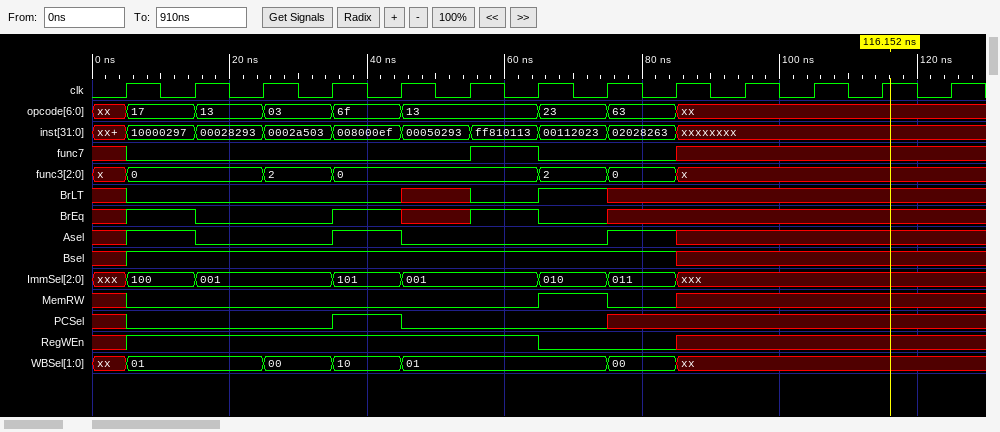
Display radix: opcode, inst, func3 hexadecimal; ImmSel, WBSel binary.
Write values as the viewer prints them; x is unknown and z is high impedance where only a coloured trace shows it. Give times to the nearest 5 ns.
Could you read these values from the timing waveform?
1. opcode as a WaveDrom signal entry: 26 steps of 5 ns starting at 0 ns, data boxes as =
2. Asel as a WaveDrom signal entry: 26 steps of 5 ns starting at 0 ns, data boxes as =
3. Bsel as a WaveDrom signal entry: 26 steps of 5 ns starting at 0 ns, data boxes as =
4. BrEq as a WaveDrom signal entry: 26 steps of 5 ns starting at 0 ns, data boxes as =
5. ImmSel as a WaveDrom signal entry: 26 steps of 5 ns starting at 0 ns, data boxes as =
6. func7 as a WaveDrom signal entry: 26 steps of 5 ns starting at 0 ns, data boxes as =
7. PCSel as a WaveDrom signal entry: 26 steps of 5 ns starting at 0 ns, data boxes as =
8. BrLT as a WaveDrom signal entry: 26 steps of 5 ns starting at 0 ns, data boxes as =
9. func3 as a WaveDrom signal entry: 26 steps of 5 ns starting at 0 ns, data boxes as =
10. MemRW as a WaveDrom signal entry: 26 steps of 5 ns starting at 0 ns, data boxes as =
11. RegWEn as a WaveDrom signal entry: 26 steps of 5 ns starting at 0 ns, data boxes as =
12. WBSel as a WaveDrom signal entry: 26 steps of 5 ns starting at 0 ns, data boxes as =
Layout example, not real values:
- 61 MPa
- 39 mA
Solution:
- {name: 'opcode', wave: 'x=.=.=.=.=...=.=.x........', data: '17 13 03 6f 13 23 63'}
- {name: 'Asel', wave: 'x1.0...1.0.....1.x........'}
- {name: 'Bsel', wave: 'x1...............x........'}
- {name: 'BrEq', wave: 'x1.0...1.x.1.0.x..........'}
- {name: 'ImmSel', wave: 'x=.=...=.=...=.=.x........', data: '100 001 101 001 010 011'}
- {name: 'func7', wave: 'x0.........1.0...x........'}
- {name: 'PCSel', wave: 'x0.....1.0.....x..........'}
- {name: 'BrLT', wave: 'x0.......x.0.1.x..........'}
- {name: 'func3', wave: 'x=...=.=.....=.=.x........', data: '0 2 0 2 0'}
- {name: 'MemRW', wave: 'x0...........1.0.x........'}
- {name: 'RegWEn', wave: 'x1...........0...x........'}
- {name: 'WBSel', wave: 'x=...=.=.=.....=.x........', data: '01 00 10 01 00'}
